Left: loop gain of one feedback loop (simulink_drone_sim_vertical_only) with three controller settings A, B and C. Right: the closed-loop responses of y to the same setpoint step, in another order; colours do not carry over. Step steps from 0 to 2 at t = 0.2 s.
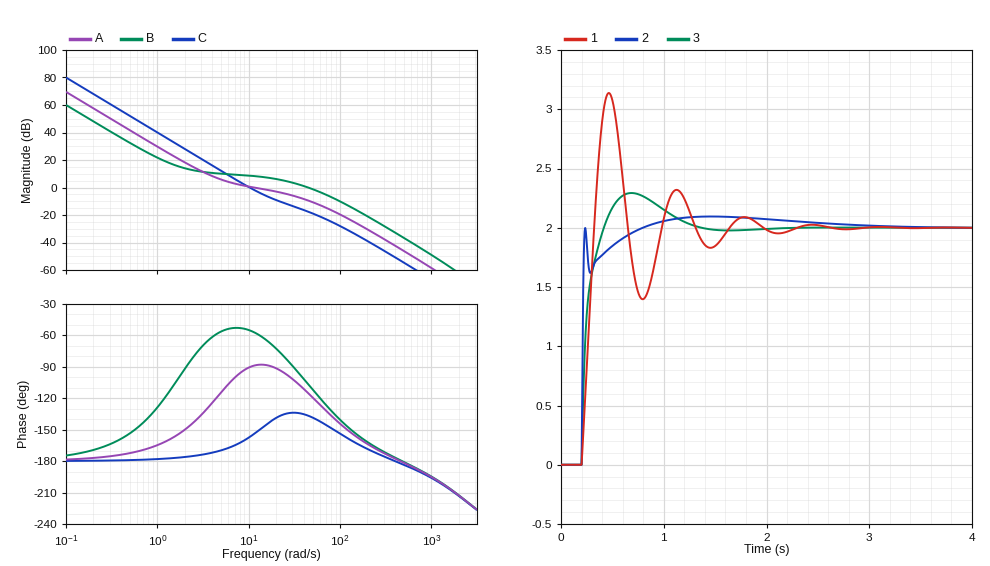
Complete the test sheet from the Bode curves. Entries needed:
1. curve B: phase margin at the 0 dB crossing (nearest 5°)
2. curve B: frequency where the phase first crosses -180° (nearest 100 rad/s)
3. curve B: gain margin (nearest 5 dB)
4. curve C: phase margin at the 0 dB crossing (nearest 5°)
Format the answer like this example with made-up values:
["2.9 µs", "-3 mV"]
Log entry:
["75°", "500 rad/s", "35 dB", "25°"]
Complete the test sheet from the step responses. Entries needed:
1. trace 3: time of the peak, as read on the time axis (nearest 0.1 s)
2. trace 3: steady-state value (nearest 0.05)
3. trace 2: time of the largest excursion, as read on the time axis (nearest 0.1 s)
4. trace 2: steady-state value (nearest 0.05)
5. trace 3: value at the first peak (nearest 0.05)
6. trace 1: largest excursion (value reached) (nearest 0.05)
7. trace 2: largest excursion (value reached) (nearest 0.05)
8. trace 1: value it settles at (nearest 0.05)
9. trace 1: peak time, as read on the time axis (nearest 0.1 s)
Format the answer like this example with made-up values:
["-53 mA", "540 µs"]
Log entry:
["0.7 s", "2.00", "1.5 s", "2.00", "2.30", "3.15", "2.10", "2.00", "0.5 s"]
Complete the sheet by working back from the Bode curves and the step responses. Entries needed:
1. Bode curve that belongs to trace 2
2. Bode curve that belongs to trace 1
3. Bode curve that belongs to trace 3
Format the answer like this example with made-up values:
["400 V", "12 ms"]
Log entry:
["B", "C", "A"]
